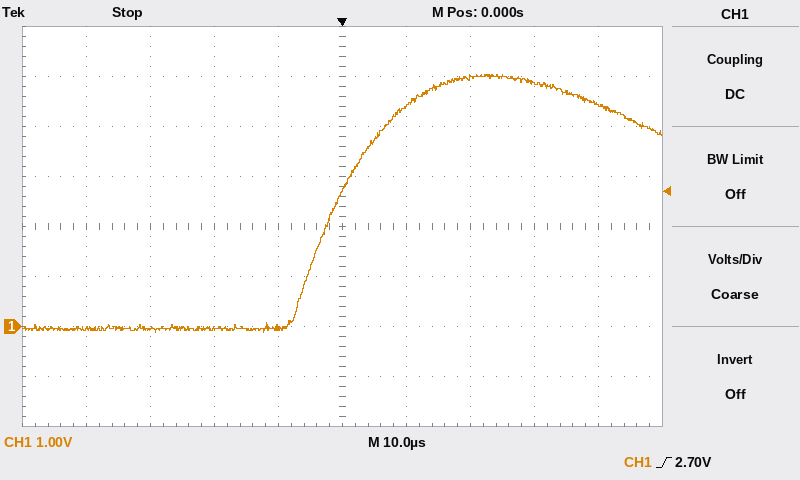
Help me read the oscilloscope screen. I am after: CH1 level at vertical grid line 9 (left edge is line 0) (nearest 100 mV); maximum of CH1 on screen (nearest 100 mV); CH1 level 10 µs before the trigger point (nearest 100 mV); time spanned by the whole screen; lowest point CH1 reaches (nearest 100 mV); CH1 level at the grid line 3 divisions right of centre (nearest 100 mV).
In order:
4.4 V
5.0 V
0.0 V
100 µs
-100 mV
4.9 V
